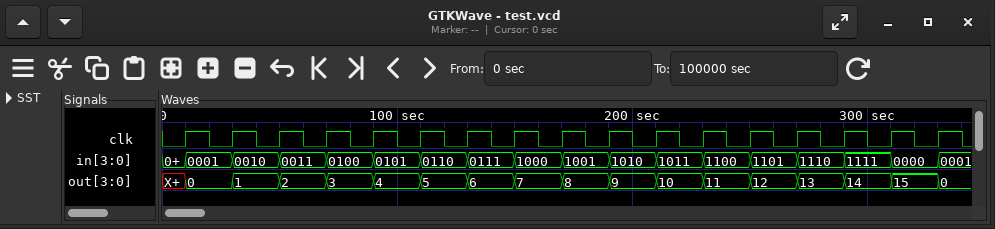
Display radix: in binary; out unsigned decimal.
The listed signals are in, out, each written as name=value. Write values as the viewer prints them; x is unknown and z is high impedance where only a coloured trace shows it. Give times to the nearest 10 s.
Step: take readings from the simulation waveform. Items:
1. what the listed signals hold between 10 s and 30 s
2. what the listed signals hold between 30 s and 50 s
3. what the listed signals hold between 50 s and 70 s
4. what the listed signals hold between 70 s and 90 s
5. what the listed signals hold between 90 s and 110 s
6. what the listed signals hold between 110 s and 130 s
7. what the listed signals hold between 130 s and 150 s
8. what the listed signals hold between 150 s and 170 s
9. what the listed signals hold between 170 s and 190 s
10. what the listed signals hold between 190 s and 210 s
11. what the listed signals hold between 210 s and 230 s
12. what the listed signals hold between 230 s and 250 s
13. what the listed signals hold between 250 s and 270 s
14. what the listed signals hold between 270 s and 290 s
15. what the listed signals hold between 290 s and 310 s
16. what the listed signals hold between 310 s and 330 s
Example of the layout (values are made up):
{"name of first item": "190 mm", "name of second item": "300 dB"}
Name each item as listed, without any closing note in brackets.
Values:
{"what the listed signals hold between 10 s and 30 s": "in=0001, out=0", "what the listed signals hold between 30 s and 50 s": "in=0010, out=1", "what the listed signals hold between 50 s and 70 s": "in=0011, out=2", "what the listed signals hold between 70 s and 90 s": "in=0100, out=3", "what the listed signals hold between 90 s and 110 s": "in=0101, out=4", "what the listed signals hold between 110 s and 130 s": "in=0110, out=5", "what the listed signals hold between 130 s and 150 s": "in=0111, out=6", "what the listed signals hold between 150 s and 170 s": "in=1000, out=7", "what the listed signals hold between 170 s and 190 s": "in=1001, out=8", "what the listed signals hold between 190 s and 210 s": "in=1010, out=9", "what the listed signals hold between 210 s and 230 s": "in=1011, out=10", "what the listed signals hold between 230 s and 250 s": "in=1100, out=11", "what the listed signals hold between 250 s and 270 s": "in=1101, out=12", "what the listed signals hold between 270 s and 290 s": "in=1110, out=13", "what the listed signals hold between 290 s and 310 s": "in=1111, out=14", "what the listed signals hold between 310 s and 330 s": "in=0000, out=15"}
